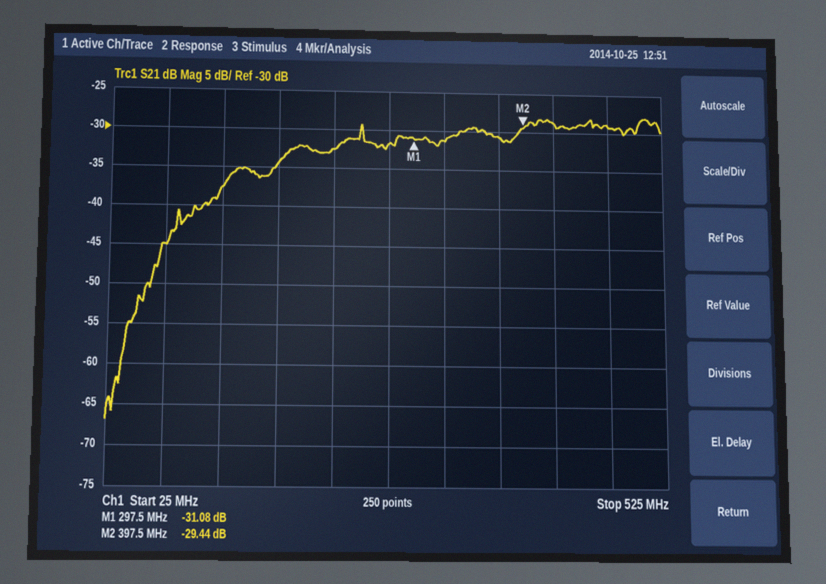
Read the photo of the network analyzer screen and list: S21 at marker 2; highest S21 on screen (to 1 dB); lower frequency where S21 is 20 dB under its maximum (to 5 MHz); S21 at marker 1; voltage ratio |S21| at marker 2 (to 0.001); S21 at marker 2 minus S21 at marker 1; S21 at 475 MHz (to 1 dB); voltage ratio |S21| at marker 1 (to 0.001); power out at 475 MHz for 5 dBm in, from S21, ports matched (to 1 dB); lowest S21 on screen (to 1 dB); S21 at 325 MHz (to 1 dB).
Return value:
-29.44 dB
-28 dB
65 MHz
-31.08 dB
0.034
1.64 dB
-29 dB
0.028
-24 dBm
-67 dB
-31 dB
